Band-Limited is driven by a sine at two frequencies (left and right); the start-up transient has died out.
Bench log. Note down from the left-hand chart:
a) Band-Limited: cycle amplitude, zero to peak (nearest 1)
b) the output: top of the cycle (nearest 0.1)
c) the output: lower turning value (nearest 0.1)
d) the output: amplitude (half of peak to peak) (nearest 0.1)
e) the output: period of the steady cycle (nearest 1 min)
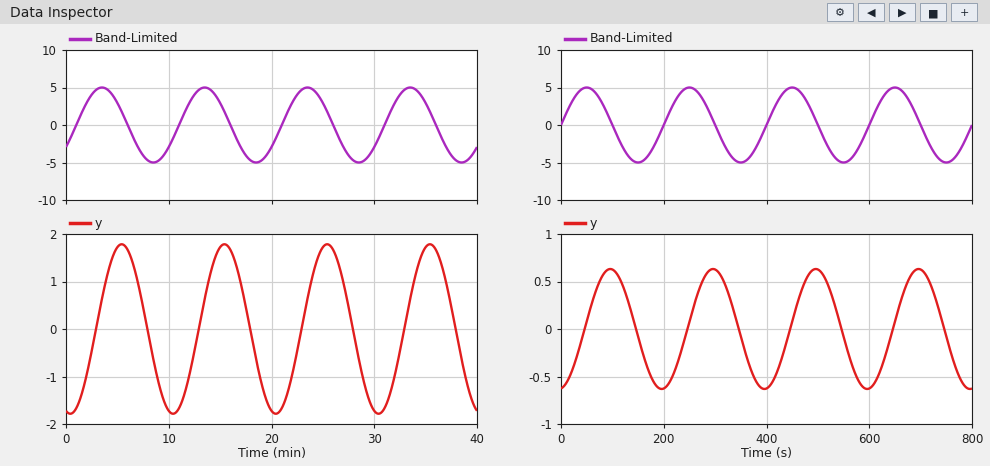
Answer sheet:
5
1.8
-1.8
1.8
10 min
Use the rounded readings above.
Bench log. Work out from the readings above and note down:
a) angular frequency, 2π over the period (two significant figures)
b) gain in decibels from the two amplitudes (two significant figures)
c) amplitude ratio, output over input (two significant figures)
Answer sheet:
0.63 rad/min
-8.9 dB
0.36
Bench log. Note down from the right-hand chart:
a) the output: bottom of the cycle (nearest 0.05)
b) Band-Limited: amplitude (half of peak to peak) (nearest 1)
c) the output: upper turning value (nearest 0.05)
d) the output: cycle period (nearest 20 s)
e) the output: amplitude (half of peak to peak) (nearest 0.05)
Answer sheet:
-0.65
5
0.65
200 s
0.65
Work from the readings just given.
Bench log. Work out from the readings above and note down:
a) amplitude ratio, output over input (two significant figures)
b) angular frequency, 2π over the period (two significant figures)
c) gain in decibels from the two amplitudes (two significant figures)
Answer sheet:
0.13
0.031 rad/s
-18 dB
